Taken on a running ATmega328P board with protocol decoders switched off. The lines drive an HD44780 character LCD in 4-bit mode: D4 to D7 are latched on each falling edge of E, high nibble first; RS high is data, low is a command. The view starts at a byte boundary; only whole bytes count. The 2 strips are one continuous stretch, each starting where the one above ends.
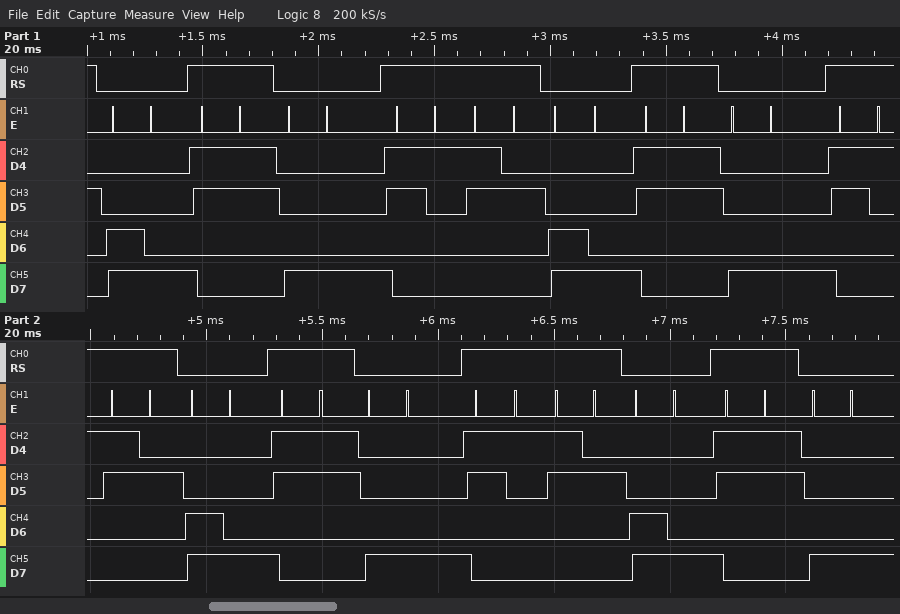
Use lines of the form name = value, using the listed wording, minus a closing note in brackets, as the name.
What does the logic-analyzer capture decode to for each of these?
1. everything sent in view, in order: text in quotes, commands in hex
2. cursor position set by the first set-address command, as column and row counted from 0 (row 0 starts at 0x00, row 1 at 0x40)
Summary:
everything sent in view, in order: text in quotes, commands in hex = 0xC8 "3" 0x88 "12" 0xC8 "3" 0x88 "12" 0xC8 "3" 0x88 "12" 0xC8 "3" 0x88
cursor position set by the first set-address command, as column and row counted from 0 = column 8, row 1
